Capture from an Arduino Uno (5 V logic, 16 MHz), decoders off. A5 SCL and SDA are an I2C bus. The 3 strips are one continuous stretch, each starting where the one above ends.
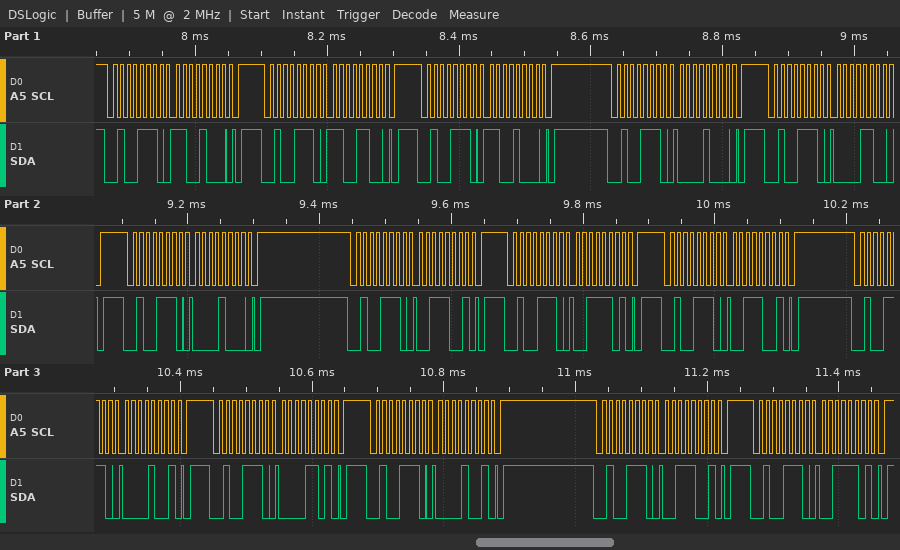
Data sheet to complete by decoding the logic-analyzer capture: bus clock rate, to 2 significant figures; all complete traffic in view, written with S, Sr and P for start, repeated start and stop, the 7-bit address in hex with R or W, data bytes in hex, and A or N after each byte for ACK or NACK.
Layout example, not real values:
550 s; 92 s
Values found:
100 kHz; S 27W A C8 A P S 27W A CC A P S 27W A C8 A P S 27W A 08 A P S 27W A 0C A P S 27W A 08 A P S 27W A 39 A P S 27W A 3D A P S 27W A 39 A P S 27W A 09 A P S 27W A 0D A P S 27W A 09 A P S 27W A 39 A P S 27W A 3D A P
